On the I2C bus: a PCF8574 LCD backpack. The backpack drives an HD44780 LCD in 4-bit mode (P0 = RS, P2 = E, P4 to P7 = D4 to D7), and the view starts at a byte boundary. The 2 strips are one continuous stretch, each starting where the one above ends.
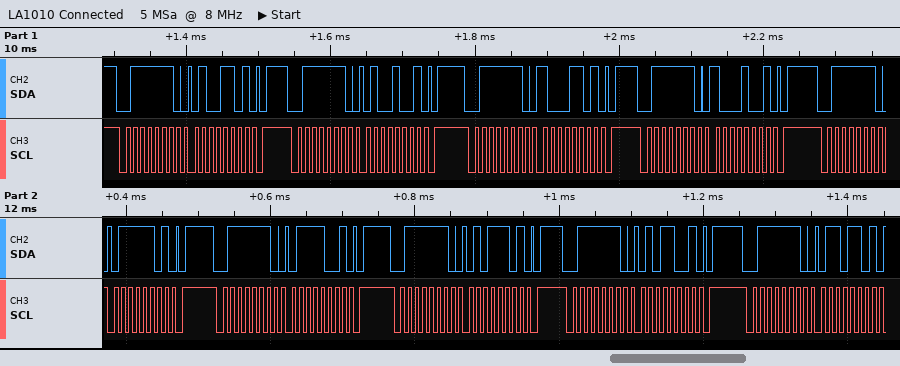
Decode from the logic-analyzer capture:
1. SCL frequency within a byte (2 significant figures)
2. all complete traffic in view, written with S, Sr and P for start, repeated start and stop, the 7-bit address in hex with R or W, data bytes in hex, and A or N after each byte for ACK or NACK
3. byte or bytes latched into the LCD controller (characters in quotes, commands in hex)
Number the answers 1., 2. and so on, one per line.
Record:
1. 100 kHz
2. S 3FW A 4D A P S 3FW A 49 A P S 3FW A 8D A P S 3FW A 89 A P S 3FW A 7D A P S 3FW A 79 A P S 3FW A 5D A P S 3FW A 59 A P S 3FW A 6D A
3. 'H' 'u'
